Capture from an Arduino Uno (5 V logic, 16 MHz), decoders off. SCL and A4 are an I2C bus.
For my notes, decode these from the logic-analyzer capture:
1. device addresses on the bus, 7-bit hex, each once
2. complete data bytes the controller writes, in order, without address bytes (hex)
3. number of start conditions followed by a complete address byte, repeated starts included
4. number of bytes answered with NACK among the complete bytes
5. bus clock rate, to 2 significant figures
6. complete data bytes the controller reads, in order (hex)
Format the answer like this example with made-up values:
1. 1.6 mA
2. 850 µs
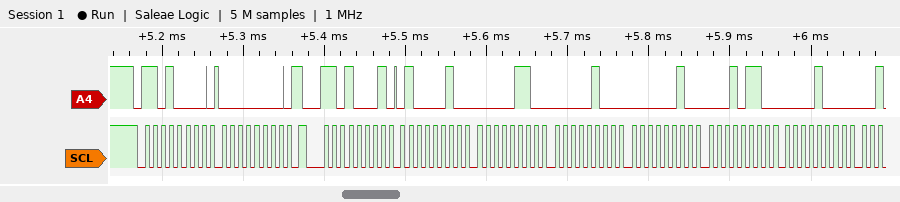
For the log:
1. 0x68
2. 00
3. 2
4. 0
5. 100 kHz
6. 42 06 04 02 16 08
